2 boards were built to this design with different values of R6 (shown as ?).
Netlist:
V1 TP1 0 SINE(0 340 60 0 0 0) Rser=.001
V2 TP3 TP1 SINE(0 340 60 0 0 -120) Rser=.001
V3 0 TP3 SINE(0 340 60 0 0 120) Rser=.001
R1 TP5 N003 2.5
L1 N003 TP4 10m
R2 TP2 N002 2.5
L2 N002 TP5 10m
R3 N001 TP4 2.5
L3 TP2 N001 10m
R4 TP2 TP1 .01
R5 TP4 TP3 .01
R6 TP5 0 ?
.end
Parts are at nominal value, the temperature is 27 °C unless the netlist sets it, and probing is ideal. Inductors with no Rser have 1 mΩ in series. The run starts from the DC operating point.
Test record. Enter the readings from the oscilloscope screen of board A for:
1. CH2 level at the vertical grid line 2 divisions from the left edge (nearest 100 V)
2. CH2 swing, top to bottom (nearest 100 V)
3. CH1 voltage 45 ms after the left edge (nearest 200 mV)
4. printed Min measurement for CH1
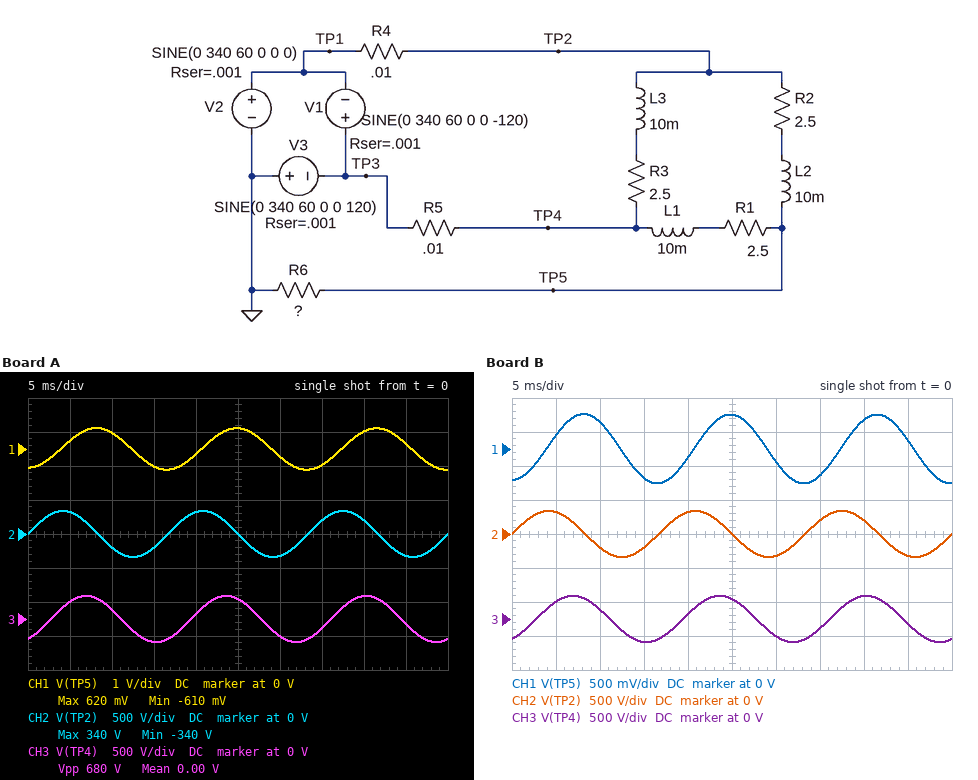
-200 V
700 V
200 mV
-610 mV
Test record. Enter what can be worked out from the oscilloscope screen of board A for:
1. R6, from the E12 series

4.7 mΩ
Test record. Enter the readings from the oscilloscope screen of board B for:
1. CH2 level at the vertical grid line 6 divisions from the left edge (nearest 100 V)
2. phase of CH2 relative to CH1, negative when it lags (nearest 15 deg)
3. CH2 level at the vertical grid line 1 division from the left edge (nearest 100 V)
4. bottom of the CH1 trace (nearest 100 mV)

-300 V
90 deg
300 V
-500 mV
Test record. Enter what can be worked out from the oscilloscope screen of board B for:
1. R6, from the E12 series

3.9 mΩ
